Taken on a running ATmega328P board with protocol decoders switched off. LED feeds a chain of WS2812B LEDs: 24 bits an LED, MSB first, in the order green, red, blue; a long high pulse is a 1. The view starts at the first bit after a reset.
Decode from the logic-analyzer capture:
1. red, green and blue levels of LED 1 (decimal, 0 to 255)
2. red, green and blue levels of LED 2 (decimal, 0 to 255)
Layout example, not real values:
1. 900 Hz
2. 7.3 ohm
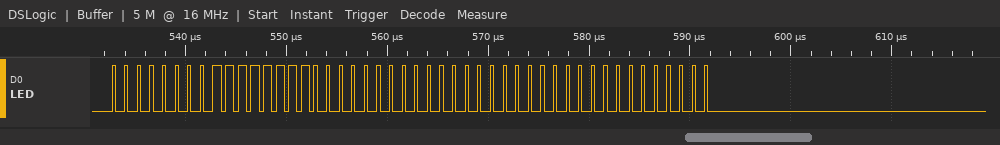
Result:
1. 255, 0, 0
2. 0, 0, 0
